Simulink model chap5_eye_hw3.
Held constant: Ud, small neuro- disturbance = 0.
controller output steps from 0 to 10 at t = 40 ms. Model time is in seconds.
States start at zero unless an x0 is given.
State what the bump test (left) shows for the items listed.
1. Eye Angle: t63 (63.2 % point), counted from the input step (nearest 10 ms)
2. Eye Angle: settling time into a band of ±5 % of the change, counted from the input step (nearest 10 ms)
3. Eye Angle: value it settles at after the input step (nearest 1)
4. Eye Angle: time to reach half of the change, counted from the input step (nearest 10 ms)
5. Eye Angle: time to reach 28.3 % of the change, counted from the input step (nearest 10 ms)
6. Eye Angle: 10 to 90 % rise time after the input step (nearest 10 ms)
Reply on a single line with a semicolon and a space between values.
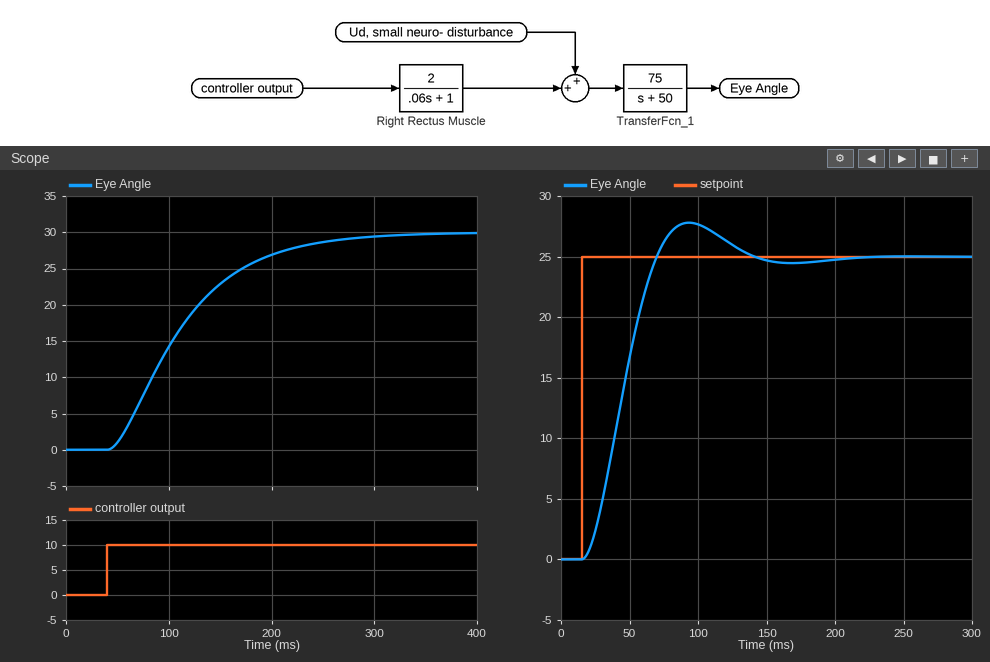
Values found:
80 ms; 200 ms; 30; 60 ms; 40 ms; 140 ms
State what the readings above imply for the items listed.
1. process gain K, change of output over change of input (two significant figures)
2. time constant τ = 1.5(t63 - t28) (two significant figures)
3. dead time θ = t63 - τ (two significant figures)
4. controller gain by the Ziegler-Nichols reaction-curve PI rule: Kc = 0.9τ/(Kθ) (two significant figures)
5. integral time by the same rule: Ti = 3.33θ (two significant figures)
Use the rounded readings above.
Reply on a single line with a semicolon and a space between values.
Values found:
3.0; 60 ms; 20 ms; 0.90; 67 ms
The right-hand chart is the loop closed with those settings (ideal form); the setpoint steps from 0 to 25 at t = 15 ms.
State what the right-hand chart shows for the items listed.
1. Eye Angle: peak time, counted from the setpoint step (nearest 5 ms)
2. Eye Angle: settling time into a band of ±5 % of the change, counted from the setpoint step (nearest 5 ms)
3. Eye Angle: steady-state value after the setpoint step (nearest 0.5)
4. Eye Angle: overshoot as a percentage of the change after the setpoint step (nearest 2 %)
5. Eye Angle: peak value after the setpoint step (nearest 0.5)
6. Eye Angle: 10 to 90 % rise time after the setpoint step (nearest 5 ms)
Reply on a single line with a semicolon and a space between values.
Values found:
80 ms; 105 ms; 25.0; 12 %; 28.0; 35 ms
